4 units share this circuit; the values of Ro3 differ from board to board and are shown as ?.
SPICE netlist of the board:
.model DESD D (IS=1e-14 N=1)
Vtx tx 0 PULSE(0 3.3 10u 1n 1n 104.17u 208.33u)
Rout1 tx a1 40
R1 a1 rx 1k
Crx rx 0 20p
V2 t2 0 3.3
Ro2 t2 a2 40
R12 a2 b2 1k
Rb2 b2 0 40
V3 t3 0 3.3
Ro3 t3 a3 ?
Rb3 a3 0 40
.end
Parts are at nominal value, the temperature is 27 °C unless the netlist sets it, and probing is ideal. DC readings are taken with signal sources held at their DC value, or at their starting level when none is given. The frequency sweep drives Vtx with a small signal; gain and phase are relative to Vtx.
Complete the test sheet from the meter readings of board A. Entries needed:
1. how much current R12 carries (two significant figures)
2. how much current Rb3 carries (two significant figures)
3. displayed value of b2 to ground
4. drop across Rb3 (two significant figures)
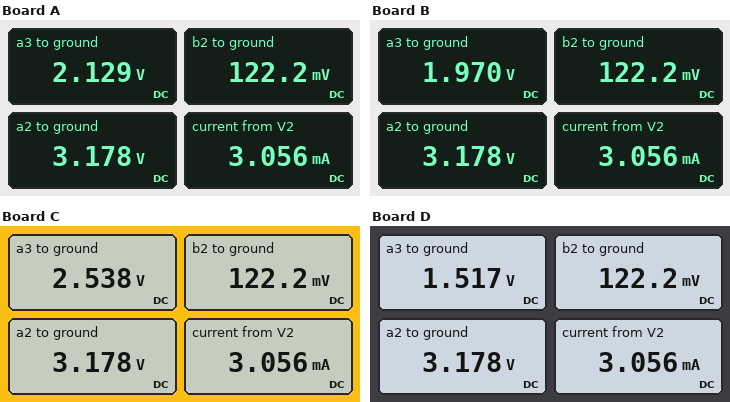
3.1 mA
53 mA
122.2 mV
2.1 V
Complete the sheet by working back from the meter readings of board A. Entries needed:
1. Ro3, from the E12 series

22 Ω
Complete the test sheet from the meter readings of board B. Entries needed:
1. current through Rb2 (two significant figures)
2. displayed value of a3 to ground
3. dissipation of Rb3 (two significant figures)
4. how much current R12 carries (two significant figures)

3.1 mA
1.970 V
97 mW
3.1 mA
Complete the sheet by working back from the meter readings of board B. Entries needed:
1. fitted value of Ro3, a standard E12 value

27 Ω
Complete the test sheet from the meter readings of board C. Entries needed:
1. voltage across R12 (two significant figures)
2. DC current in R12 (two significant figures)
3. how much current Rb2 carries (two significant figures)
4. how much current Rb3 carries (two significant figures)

3.1 V
3.1 mA
3.1 mA
63 mA
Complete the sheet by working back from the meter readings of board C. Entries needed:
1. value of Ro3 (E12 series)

12 Ω
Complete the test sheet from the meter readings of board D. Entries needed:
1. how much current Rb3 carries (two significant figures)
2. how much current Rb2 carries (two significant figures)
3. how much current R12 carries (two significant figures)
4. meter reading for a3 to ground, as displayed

38 mA
3.1 mA
3.1 mA
1.517 V
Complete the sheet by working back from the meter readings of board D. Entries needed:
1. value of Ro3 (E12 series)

47 Ω
